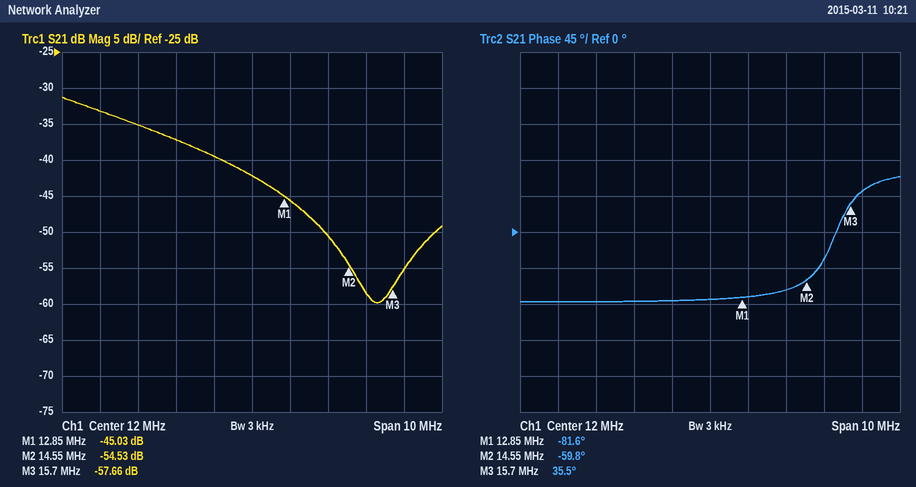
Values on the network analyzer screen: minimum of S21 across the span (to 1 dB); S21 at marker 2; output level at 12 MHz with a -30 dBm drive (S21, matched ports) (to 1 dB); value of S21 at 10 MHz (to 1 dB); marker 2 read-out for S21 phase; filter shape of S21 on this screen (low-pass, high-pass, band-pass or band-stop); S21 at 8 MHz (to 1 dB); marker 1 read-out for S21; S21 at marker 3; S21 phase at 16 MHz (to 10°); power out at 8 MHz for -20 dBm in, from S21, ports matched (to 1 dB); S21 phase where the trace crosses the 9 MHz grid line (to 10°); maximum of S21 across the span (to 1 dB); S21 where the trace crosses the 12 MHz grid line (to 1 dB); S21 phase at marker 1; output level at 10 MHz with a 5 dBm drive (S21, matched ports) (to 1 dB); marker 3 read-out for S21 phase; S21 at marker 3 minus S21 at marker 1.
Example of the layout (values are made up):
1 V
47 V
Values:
-60 dB
-54.53 dB
-72 dBm
-37 dB
-59.8°
low-pass
-33 dB
-45.03 dB
-57.66 dB
50°
-53 dBm
-90°
-31 dB
-42 dB
-81.6°
-32 dBm
35.5°
-12.63 dB
